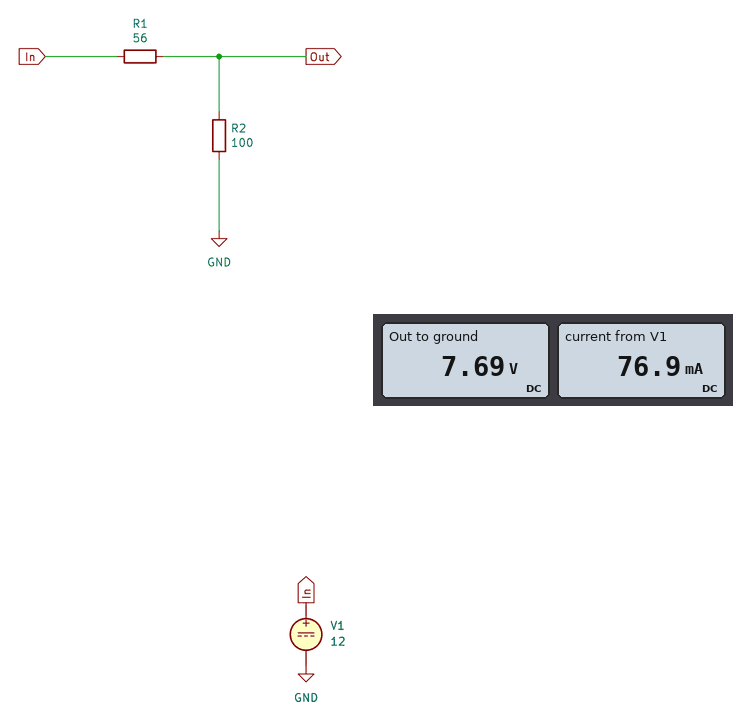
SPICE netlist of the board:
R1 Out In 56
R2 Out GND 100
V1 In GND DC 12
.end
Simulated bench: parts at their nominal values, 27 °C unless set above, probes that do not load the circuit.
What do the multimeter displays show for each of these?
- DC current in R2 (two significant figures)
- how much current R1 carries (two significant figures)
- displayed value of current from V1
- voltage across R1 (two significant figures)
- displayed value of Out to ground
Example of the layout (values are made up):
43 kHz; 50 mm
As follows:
77 mA; 77 mA; 76.9 mA; 4.3 V; 7.69 V
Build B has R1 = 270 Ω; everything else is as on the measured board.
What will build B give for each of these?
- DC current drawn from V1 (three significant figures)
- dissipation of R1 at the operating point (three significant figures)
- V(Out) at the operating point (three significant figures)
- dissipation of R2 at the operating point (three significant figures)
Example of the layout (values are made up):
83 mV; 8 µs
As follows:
32.4 mA; 284 mW; 3.24 V; 105 mW
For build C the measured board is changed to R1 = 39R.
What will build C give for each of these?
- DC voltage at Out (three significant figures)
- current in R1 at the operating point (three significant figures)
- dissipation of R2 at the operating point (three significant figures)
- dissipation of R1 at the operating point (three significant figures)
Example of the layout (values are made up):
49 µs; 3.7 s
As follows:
8.63 V; 86.3 mA; 745 mW; 291 mW
